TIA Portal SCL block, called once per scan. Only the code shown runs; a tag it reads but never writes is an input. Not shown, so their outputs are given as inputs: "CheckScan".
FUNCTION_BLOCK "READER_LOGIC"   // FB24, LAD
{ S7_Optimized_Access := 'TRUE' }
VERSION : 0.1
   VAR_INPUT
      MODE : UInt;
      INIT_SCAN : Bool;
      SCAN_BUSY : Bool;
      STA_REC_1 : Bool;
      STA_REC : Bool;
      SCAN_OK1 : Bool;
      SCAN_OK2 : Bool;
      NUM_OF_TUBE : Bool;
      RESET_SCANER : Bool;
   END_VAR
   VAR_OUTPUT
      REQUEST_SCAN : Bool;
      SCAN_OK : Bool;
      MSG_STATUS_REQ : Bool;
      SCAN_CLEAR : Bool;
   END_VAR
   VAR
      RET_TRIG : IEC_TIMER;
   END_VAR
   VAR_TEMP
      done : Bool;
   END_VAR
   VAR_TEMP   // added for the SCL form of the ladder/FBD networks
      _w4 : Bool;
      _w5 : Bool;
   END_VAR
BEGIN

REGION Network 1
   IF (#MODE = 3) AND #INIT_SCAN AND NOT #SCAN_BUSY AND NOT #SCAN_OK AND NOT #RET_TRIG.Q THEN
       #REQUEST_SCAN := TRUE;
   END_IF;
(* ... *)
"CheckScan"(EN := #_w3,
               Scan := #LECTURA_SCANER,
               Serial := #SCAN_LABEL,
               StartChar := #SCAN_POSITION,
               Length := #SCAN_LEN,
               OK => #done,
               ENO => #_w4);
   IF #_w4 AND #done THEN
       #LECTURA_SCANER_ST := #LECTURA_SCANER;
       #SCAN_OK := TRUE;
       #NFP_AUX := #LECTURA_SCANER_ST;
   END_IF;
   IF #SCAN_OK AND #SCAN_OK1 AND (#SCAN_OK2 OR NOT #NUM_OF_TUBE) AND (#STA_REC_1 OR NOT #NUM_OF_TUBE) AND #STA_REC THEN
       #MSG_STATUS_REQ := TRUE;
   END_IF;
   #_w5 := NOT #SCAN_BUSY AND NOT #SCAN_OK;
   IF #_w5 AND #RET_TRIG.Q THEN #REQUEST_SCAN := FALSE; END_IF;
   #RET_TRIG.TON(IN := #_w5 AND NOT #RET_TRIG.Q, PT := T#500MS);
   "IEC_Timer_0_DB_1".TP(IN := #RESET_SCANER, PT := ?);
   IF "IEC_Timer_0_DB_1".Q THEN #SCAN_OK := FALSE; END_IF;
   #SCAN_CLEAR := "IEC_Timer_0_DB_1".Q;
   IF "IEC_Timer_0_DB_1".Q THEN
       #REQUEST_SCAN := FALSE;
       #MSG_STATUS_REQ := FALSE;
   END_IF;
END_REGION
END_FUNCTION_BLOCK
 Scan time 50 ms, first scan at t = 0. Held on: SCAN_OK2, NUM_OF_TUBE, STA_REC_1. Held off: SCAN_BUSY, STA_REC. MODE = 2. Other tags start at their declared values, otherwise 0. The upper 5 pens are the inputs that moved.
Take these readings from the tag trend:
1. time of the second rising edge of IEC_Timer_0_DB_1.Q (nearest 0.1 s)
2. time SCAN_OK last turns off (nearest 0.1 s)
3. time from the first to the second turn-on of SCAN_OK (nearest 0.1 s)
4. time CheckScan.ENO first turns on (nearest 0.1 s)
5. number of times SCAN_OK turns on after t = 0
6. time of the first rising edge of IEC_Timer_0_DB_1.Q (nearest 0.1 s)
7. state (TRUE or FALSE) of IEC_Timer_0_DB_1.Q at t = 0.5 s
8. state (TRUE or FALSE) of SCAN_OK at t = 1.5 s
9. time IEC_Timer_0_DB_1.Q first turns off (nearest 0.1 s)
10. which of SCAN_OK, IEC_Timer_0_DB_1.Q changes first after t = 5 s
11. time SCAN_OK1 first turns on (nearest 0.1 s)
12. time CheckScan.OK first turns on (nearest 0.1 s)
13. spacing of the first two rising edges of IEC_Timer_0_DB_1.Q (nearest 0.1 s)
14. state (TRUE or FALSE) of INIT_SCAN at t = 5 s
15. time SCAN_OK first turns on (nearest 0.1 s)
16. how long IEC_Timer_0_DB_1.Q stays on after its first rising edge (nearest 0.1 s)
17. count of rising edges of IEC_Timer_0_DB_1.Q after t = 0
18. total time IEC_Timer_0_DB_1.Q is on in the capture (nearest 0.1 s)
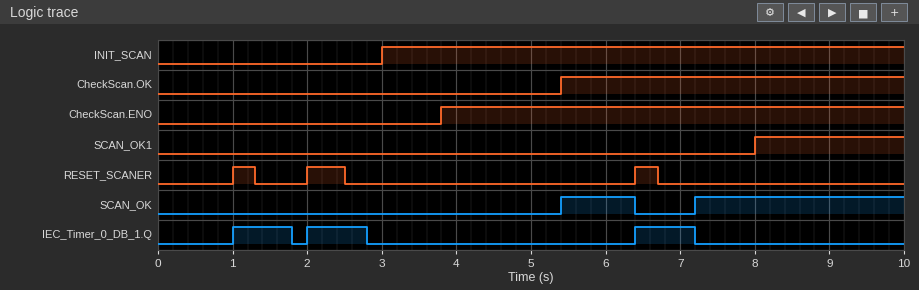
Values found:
2.0 s
6.4 s
1.8 s
3.8 s
2
1.0 s
FALSE
FALSE
1.8 s
SCAN_OK
8.0 s
5.4 s
1.0 s
TRUE
5.4 s
0.8 s
3
2.4 s
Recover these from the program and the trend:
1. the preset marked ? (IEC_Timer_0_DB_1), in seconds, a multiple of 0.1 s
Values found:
0.8 s
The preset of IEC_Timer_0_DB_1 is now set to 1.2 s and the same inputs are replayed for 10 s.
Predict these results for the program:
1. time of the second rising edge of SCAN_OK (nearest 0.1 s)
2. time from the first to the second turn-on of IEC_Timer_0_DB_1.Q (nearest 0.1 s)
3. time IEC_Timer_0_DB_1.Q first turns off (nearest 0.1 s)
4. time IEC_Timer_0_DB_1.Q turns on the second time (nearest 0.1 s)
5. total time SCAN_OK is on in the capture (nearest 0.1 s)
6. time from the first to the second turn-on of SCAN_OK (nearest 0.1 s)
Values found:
7.6 s
5.4 s
2.2 s
6.4 s
3.4 s
2.2 s
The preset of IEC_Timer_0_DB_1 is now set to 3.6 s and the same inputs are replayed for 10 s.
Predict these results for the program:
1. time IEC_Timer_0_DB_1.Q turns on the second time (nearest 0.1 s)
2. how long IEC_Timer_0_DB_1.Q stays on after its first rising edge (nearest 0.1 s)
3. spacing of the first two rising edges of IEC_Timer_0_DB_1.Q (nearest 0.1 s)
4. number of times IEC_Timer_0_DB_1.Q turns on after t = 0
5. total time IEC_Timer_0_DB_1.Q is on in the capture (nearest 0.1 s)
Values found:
6.4 s
3.6 s
5.4 s
2
7.2 s
